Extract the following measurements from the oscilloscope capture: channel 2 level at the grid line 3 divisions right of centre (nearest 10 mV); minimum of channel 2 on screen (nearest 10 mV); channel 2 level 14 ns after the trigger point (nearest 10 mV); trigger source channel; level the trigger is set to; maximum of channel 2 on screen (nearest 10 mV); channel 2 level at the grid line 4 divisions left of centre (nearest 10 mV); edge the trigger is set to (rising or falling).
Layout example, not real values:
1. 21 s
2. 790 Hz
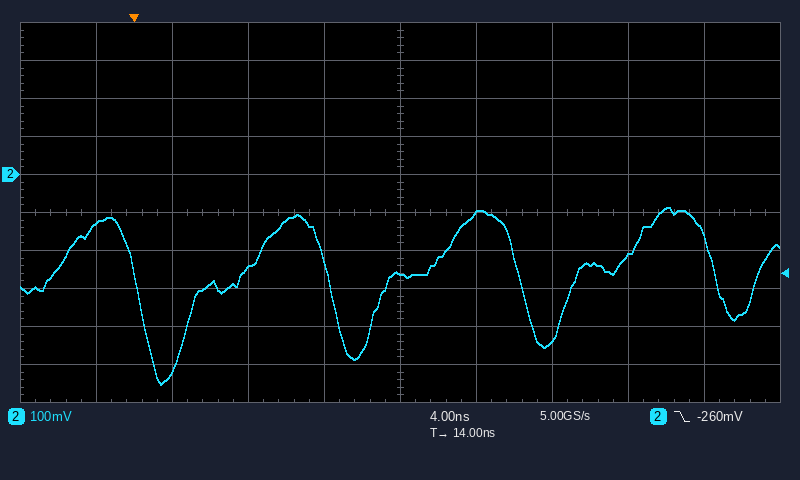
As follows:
1. -220 mV
2. -550 mV
3. -260 mV
4. channel 2
5. -260 mV
6. -90 mV
7. -130 mV
8. falling
